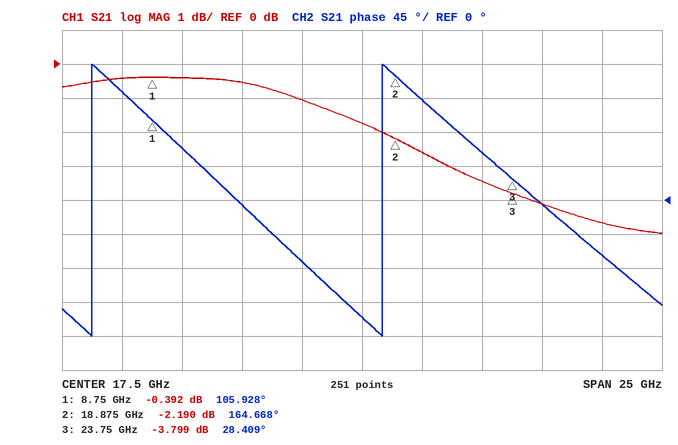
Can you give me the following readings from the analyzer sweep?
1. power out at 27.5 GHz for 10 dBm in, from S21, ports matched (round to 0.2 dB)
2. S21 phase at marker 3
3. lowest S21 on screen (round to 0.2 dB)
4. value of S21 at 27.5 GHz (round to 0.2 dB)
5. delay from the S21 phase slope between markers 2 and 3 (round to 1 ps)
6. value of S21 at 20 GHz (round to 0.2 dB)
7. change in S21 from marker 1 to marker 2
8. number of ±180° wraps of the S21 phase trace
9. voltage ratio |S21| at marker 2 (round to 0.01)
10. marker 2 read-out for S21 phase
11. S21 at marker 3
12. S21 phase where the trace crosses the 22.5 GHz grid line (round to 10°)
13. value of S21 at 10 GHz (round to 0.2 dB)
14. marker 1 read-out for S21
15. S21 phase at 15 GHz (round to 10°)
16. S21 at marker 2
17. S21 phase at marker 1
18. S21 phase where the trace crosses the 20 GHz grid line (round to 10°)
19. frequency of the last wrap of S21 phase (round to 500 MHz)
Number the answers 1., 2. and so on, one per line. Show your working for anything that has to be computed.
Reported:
1. 10 dBm + (-4.6 dB) = 5.4 dBm
2. 28.409°
3. -5.0 dB
4. -4.6 dB
5. −(28.409° − (164.668°))/(360° × 4.875 GHz) ≈ 78 ps
6. -2.6 dB
7. -2.19 − (-0.392) = -1.798 dB
8. 2
9. 10^(-2.19/20) ≈ 0.78
10. 164.668°
11. -3.799 dB
12. 60°
13. -0.4 dB
14. -0.392 dB
15. -80°
16. -2.190 dB
17. 105.928°
18. 130°
19. 18.5 GHz
